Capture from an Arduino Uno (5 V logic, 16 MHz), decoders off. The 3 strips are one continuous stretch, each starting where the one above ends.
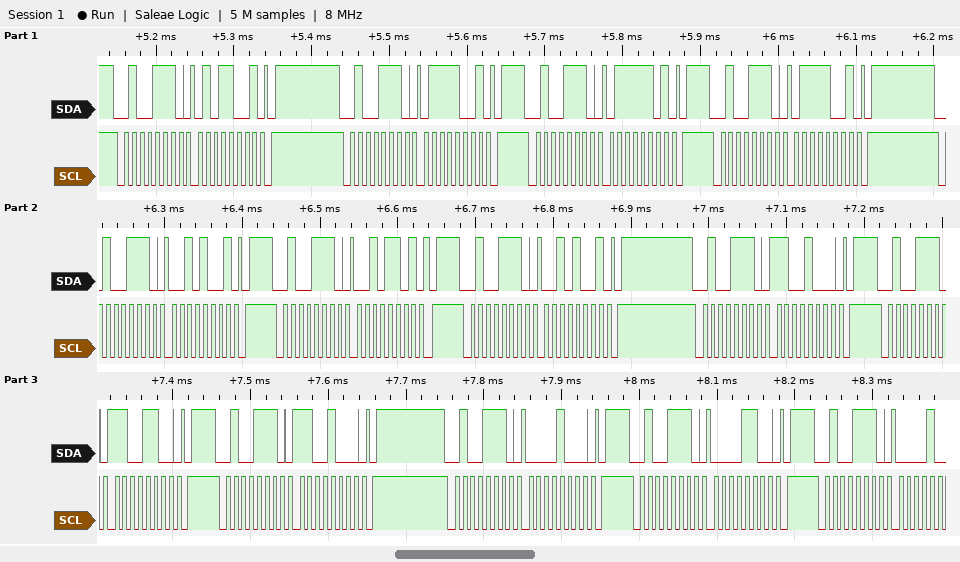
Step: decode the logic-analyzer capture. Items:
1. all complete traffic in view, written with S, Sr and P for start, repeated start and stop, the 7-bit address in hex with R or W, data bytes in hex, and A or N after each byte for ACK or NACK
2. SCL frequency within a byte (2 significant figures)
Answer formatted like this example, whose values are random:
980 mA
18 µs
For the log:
S 27W A 59 A P S 27W A 79 A P S 27W A 7D A P S 27W A 79 A P S 27W A 29 A P S 27W A 2D A P S 27W A 29 A P S 27W A C8 A P S 27W A CC A P S 27W A C8 A P S 27W A 08 A P S 27W A 0C A P S 27W A
100 kHz
